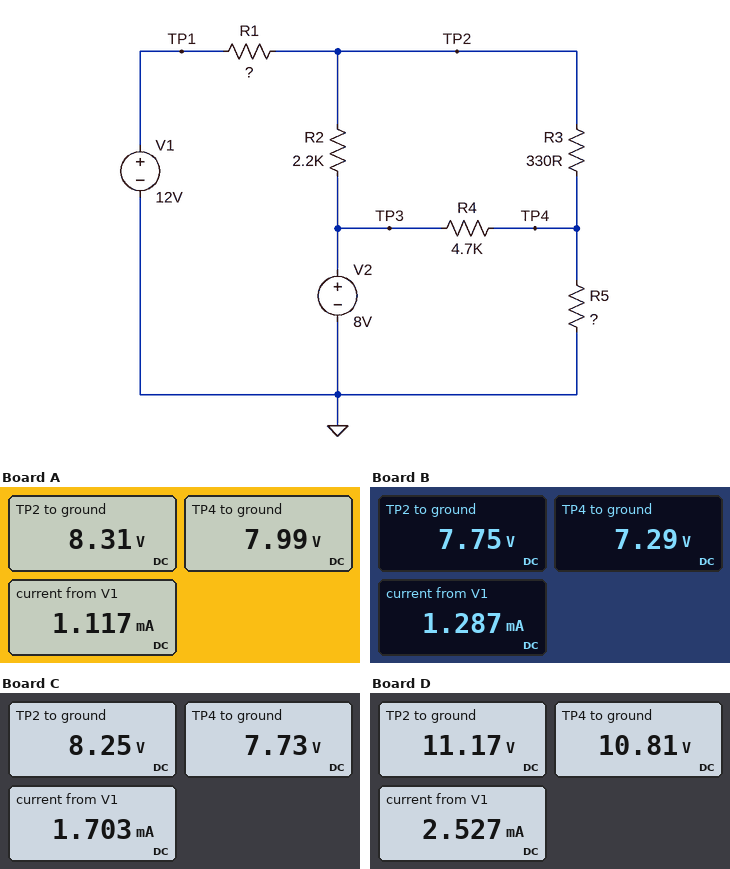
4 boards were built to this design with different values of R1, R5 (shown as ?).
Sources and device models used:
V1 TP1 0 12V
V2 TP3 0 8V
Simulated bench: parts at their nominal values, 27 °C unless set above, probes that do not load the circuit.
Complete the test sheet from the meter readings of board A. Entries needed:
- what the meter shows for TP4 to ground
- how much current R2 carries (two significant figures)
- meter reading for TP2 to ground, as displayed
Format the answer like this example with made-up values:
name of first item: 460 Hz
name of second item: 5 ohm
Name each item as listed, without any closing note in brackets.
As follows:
what the meter shows for TP4 to ground: 7.99 V
how much current R2 carries: 140 µA
meter reading for TP2 to ground, as displayed: 8.31 V
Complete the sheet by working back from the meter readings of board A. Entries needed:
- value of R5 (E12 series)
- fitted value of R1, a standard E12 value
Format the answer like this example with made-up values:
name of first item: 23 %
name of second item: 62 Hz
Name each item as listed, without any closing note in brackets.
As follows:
value of R5: 8.2 kΩ
fitted value of R1, a standard E12 value: 3.3 kΩ
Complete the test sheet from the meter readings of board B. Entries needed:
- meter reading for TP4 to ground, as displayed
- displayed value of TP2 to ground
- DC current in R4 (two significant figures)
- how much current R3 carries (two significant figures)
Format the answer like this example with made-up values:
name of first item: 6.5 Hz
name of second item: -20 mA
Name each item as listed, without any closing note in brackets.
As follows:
meter reading for TP4 to ground, as displayed: 7.29 V
displayed value of TP2 to ground: 7.75 V
DC current in R4: 150 µA
how much current R3 carries: 1.4 mA
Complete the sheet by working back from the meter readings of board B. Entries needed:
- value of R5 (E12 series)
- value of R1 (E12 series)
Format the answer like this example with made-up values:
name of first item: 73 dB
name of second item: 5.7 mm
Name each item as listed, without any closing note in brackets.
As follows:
value of R5: 4.7 kΩ
value of R1: 3.3 kΩ
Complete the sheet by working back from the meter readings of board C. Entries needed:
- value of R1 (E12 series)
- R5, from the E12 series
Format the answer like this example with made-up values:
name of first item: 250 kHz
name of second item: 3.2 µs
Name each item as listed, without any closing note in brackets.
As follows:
value of R1: 2.2 kΩ
R5, from the E12 series: 4.7 kΩ
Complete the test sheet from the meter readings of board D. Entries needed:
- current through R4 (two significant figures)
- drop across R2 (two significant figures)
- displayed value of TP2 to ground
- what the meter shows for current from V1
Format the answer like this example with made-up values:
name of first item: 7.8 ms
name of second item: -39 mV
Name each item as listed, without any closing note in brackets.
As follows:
current through R4: 600 µA
drop across R2: 3.2 V
displayed value of TP2 to ground: 11.17 V
what the meter shows for current from V1: 2.527 mA
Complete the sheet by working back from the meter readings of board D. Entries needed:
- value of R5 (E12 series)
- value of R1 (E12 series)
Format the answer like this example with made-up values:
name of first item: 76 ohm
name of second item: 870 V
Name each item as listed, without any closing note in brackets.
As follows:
value of R5: 22 kΩ
value of R1: 330 Ω
